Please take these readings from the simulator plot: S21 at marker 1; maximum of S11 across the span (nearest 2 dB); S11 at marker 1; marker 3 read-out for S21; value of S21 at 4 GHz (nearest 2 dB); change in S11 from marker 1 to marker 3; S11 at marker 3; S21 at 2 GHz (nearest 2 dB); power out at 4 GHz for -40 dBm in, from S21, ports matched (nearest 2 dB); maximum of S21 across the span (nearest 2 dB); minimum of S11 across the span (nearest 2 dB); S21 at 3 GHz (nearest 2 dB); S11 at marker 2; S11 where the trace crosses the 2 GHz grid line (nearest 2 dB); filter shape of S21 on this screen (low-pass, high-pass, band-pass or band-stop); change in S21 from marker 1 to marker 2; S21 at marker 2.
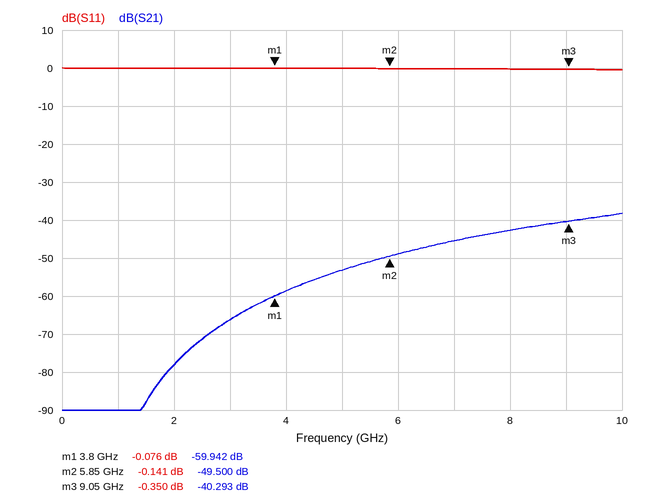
-59.942 dB
0 dB
-0.076 dB
-40.293 dB
-58 dB
-0.274 dB
-0.350 dB
-78 dB
-98 dBm
-38 dB
0 dB
-66 dB
-0.141 dB
0 dB
high-pass
10.442 dB
-49.500 dB
